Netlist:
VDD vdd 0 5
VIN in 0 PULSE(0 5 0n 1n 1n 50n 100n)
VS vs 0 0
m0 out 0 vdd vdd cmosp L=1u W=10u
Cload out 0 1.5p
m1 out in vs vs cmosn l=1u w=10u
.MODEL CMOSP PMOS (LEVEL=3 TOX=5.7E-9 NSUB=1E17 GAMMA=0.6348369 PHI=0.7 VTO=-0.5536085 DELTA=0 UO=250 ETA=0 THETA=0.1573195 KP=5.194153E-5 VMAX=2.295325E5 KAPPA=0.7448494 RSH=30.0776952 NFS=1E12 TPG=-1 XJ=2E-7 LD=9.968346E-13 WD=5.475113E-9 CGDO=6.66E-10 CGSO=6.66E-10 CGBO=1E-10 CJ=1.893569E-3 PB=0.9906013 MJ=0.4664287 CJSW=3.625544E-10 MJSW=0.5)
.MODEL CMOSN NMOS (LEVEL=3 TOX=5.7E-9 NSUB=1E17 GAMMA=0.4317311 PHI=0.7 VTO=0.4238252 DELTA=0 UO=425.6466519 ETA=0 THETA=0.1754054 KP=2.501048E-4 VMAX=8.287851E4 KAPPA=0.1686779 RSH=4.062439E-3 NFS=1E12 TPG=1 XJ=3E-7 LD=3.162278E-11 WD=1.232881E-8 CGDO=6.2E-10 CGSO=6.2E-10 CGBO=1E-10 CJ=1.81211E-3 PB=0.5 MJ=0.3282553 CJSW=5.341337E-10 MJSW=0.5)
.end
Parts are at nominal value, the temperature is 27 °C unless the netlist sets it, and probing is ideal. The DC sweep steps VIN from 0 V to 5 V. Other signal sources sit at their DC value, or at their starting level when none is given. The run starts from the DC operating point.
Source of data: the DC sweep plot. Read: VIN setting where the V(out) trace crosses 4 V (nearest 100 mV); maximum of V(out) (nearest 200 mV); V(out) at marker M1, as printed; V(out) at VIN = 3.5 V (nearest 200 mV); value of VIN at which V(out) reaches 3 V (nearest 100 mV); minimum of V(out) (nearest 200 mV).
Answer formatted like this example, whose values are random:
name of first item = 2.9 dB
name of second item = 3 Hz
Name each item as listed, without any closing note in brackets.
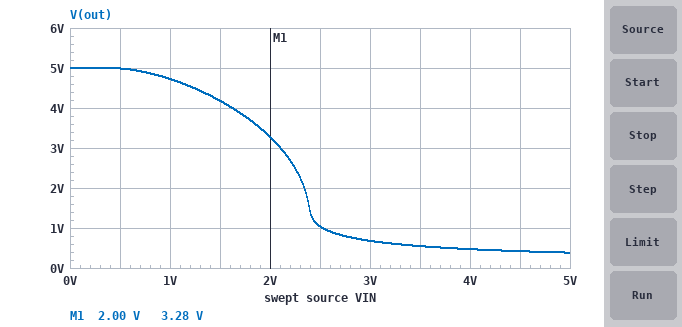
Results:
VIN setting where the V(out) trace crosses 4 V = 1.6 V
maximum of V(out) = 5.0 V
V(out) at marker M1, as printed = 3.28 V
V(out) at VIN = 3.5 V = 600 mV
value of VIN at which V(out) reaches 3 V = 2.1 V
minimum of V(out) = 400 mV
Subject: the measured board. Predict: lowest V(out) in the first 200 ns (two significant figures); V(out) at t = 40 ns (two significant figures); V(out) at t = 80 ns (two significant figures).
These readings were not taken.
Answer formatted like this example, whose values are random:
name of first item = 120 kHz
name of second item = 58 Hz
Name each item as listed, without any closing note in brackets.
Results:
lowest V(out) in the first 200 ns = 380 mV
V(out) at t = 40 ns = 380 mV
V(out) at t = 80 ns = 5.0 V
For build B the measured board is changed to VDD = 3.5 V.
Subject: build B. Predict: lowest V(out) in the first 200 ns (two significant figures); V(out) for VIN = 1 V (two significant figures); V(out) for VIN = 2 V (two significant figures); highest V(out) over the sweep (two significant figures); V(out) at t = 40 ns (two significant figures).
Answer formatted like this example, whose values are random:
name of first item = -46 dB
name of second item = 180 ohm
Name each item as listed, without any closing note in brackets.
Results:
lowest V(out) in the first 200 ns = 180 mV
V(out) for VIN = 1 V = 3.1 V
V(out) for VIN = 2 V = 530 mV
highest V(out) over the sweep = 3.5 V
V(out) at t = 40 ns = 190 mV
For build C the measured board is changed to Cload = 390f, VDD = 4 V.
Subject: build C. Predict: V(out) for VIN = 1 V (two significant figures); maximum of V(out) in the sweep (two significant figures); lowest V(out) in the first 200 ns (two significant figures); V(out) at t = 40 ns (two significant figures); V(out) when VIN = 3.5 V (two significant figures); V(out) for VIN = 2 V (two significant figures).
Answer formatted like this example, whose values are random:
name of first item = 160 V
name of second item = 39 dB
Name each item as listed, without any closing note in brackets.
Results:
V(out) for VIN = 1 V = 3.7 V
maximum of V(out) in the sweep = 4.0 V
lowest V(out) in the first 200 ns = 230 mV
V(out) at t = 40 ns = 250 mV
V(out) when VIN = 3.5 V = 340 mV
V(out) for VIN = 2 V = 900 mV
